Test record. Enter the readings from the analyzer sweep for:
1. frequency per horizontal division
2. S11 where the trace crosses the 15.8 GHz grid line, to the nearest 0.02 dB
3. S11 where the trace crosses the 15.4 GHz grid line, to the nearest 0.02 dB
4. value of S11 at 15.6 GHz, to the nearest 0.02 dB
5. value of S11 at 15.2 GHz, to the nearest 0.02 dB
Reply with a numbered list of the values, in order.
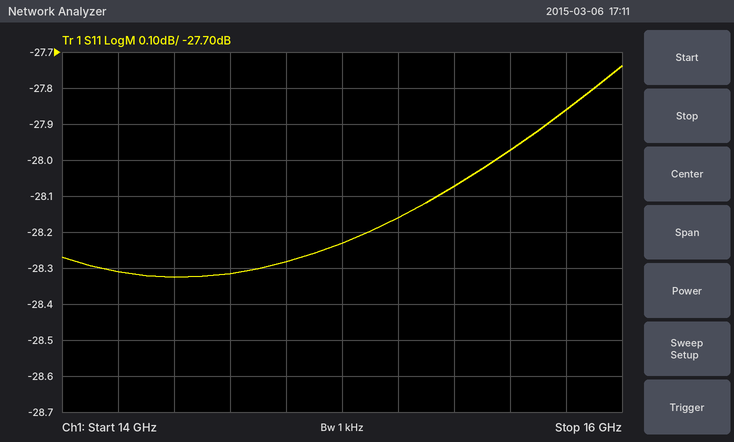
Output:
1. 200 MHz
2. -27.86 dB
3. -28.08 dB
4. -27.98 dB
5. -28.16 dB
